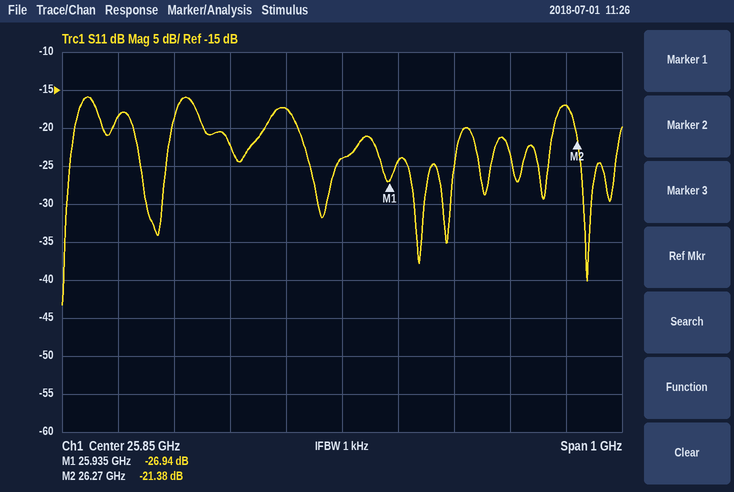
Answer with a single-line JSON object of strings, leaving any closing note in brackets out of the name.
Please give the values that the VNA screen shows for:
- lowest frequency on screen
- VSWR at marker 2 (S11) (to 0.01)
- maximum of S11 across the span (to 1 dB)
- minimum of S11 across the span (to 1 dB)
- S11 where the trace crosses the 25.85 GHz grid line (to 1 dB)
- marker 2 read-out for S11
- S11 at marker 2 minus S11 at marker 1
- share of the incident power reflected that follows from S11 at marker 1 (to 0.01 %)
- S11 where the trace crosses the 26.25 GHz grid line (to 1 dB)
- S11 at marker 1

{"lowest frequency on screen": "25.35 GHz", "VSWR at marker 2 (S11)": "1.19", "maximum of S11 across the span": "-16 dB", "minimum of S11 across the span": "-43 dB", "S11 where the trace crosses the 25.85 GHz grid line": "-24 dB", "marker 2 read-out for S11": "-21.38 dB", "S11 at marker 2 minus S11 at marker 1": "5.56 dB", "share of the incident power reflected that follows from S11 at marker 1": "0.20 %", "S11 where the trace crosses the 26.25 GHz grid line": "-17 dB", "S11 at marker 1": "-26.94 dB"}
